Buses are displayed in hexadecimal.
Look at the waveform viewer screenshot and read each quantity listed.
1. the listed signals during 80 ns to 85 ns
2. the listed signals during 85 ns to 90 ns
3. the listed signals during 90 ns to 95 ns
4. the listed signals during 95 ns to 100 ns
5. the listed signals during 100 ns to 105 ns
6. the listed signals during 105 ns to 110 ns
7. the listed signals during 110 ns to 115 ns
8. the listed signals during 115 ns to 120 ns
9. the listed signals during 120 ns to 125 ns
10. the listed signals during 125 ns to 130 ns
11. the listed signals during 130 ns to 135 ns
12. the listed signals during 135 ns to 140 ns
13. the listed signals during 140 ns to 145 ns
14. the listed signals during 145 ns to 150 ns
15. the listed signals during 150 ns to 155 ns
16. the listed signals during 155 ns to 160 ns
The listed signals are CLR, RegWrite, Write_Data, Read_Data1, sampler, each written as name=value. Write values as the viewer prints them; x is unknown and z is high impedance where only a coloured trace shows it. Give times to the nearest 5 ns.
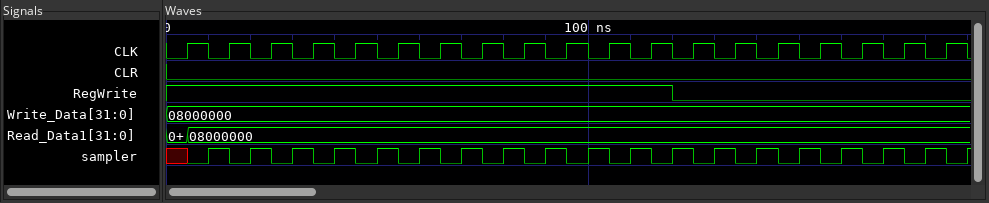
CLR=0, RegWrite=1, Write_Data=08000000, Read_Data1=08000000, sampler=1
CLR=0, RegWrite=1, Write_Data=08000000, Read_Data1=08000000, sampler=0
CLR=0, RegWrite=1, Write_Data=08000000, Read_Data1=08000000, sampler=1
CLR=0, RegWrite=1, Write_Data=08000000, Read_Data1=08000000, sampler=0
CLR=0, RegWrite=1, Write_Data=08000000, Read_Data1=08000000, sampler=1
CLR=0, RegWrite=1, Write_Data=08000000, Read_Data1=08000000, sampler=0
CLR=0, RegWrite=1, Write_Data=08000000, Read_Data1=08000000, sampler=1
CLR=0, RegWrite=1, Write_Data=08000000, Read_Data1=08000000, sampler=0
CLR=0, RegWrite=0, Write_Data=08000000, Read_Data1=08000000, sampler=1
CLR=0, RegWrite=0, Write_Data=08000000, Read_Data1=08000000, sampler=0
CLR=0, RegWrite=0, Write_Data=08000000, Read_Data1=08000000, sampler=1
CLR=0, RegWrite=0, Write_Data=08000000, Read_Data1=08000000, sampler=0
CLR=0, RegWrite=0, Write_Data=08000000, Read_Data1=08000000, sampler=1
CLR=0, RegWrite=0, Write_Data=08000000, Read_Data1=08000000, sampler=0
CLR=0, RegWrite=0, Write_Data=08000000, Read_Data1=08000000, sampler=1
CLR=0, RegWrite=0, Write_Data=08000000, Read_Data1=08000000, sampler=0
